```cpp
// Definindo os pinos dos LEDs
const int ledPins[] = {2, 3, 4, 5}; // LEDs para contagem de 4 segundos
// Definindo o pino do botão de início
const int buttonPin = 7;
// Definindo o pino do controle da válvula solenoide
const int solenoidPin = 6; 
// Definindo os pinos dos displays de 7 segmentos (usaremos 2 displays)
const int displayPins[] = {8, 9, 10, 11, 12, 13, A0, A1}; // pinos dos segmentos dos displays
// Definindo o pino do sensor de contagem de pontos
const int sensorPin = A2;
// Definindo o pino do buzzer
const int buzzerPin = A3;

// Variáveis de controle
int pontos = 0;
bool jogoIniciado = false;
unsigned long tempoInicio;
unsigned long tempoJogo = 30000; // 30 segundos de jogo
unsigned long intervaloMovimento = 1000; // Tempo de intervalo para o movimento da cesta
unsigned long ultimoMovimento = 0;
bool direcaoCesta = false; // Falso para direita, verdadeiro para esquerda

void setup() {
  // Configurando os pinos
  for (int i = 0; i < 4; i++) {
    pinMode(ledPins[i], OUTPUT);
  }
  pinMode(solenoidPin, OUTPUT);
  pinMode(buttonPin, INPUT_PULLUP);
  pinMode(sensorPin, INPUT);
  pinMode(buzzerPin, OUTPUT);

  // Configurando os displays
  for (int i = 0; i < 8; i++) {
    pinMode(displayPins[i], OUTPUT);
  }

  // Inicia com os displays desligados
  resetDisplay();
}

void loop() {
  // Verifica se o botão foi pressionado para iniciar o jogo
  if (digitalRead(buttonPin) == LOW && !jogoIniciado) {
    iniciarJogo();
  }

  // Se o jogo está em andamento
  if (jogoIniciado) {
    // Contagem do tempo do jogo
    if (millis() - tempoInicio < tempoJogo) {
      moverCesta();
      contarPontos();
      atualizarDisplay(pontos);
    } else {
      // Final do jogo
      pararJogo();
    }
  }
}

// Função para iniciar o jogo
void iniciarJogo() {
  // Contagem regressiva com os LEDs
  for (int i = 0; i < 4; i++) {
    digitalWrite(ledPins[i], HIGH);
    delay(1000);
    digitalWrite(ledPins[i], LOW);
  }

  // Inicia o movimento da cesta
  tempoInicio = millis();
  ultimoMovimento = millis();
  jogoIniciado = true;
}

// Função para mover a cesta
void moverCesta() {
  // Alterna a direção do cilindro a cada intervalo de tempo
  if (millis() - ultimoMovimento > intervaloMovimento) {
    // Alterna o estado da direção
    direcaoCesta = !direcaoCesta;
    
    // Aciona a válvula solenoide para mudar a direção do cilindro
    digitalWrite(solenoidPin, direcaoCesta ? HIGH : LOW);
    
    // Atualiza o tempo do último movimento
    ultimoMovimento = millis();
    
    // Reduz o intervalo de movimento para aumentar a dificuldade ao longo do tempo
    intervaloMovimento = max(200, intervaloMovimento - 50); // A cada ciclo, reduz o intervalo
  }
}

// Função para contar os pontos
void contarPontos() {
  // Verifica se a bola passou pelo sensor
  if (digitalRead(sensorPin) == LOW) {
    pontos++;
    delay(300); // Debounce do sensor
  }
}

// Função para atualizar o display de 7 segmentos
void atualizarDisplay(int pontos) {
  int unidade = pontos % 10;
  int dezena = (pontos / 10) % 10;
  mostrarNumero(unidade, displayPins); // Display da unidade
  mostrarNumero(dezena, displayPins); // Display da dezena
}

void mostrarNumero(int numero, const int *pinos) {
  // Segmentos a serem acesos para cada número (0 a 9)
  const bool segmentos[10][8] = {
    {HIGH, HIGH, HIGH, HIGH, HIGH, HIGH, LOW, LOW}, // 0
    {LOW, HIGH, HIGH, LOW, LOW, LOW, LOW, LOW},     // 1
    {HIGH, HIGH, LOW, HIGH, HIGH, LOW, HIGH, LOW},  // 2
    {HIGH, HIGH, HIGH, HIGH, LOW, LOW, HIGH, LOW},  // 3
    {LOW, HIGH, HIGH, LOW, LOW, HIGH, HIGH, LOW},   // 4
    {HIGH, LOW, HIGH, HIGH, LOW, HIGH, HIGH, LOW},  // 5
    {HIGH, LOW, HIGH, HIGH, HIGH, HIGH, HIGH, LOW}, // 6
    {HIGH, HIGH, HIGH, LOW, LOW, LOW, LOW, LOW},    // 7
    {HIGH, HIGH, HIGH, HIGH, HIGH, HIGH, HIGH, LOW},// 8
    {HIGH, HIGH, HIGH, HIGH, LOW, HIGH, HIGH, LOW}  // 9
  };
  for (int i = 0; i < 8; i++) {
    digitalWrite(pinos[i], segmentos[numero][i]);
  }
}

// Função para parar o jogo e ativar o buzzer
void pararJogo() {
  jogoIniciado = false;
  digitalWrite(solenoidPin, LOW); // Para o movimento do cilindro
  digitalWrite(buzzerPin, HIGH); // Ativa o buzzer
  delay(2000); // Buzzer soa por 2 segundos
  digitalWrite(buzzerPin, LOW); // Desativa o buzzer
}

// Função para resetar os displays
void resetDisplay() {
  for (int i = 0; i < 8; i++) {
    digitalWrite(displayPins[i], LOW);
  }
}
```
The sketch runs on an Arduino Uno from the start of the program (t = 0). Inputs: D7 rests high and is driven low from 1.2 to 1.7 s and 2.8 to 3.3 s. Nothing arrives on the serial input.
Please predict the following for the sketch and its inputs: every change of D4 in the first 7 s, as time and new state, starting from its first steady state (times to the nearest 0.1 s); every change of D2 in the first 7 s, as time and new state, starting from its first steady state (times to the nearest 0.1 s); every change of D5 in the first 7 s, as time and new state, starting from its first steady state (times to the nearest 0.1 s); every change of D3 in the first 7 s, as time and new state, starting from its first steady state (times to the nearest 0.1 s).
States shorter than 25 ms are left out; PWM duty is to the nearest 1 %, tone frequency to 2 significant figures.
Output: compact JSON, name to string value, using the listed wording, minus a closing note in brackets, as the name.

{"every change of D4 in the first 7 s, as time and new state, starting from its first steady state": "0 s low; 3.2 s high; 4.2 s low", "every change of D2 in the first 7 s, as time and new state, starting from its first steady state": "0 s low; 1.2 s high; 2.2 s low", "every change of D5 in the first 7 s, as time and new state, starting from its first steady state": "0 s low; 4.2 s high; 5.2 s low", "every change of D3 in the first 7 s, as time and new state, starting from its first steady state": "0 s low; 2.2 s high; 3.2 s low"}
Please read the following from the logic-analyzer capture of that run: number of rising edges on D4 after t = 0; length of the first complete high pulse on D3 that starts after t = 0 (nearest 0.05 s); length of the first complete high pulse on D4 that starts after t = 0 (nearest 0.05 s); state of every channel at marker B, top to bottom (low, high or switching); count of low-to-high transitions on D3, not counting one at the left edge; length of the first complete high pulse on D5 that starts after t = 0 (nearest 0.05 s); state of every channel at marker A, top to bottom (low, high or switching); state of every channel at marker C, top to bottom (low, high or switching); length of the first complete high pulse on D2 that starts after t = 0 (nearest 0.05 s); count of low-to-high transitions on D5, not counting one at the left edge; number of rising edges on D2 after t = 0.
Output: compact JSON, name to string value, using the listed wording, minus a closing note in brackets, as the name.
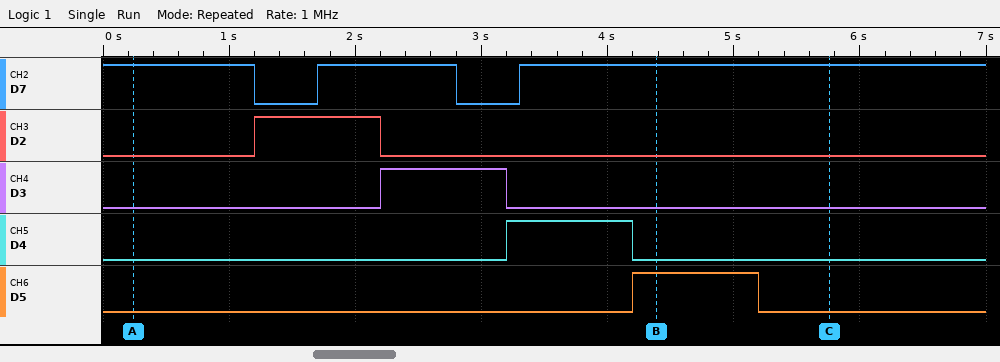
{"number of rising edges on D4 after t = 0": "1", "length of the first complete high pulse on D3 that starts after t = 0": "1.00 s", "length of the first complete high pulse on D4 that starts after t = 0": "1.00 s", "state of every channel at marker B, top to bottom": "D7 high, D2 low, D3 low, D4 low, D5 high", "count of low-to-high transitions on D3, not counting one at the left edge": "1", "length of the first complete high pulse on D5 that starts after t = 0": "1.00 s", "state of every channel at marker A, top to bottom": "D7 high, D2 low, D3 low, D4 low, D5 low", "state of every channel at marker C, top to bottom": "D7 high, D2 low, D3 low, D4 low, D5 low", "length of the first complete high pulse on D2 that starts after t = 0": "1.00 s", "count of low-to-high transitions on D5, not counting one at the left edge": "1", "number of rising edges on D2 after t = 0": "1"}
